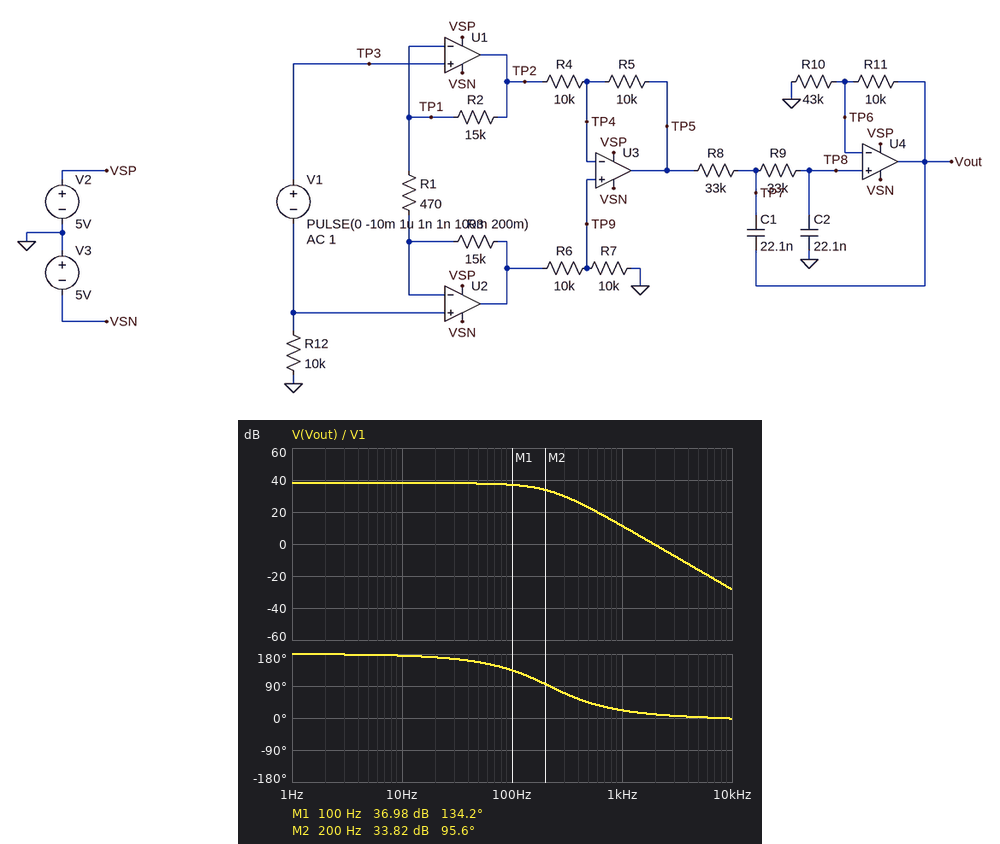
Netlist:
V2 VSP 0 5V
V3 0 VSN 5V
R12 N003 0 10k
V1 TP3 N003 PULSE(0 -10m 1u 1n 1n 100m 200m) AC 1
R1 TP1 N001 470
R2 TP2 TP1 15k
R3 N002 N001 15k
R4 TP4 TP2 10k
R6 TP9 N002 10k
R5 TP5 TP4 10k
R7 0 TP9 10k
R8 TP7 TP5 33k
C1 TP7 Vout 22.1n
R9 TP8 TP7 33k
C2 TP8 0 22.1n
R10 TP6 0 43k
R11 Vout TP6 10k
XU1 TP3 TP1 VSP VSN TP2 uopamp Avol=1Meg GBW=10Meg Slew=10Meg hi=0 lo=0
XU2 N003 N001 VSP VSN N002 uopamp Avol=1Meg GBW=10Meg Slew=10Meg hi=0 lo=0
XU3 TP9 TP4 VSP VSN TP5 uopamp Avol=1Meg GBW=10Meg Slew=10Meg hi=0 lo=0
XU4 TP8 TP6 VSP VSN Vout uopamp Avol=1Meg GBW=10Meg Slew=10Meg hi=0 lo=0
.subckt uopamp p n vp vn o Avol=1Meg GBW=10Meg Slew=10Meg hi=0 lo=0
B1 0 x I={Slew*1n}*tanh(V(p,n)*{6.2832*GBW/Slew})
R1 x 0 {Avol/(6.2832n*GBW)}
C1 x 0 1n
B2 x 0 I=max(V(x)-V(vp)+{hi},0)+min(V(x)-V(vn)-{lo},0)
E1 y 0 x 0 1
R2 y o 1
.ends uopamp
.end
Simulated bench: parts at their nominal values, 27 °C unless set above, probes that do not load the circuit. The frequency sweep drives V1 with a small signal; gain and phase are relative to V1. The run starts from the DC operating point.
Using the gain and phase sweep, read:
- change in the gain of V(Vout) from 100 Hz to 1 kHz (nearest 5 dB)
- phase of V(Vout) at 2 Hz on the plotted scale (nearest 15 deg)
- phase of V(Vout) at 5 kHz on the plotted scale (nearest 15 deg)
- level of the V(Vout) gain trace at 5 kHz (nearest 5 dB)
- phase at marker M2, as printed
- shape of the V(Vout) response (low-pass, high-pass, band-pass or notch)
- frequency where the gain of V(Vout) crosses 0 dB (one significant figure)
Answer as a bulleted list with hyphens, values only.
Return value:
- -25 dB
- 180 deg
- 0 deg
- -15 dB
- 95.6 deg
- low-pass
- 2 kHz
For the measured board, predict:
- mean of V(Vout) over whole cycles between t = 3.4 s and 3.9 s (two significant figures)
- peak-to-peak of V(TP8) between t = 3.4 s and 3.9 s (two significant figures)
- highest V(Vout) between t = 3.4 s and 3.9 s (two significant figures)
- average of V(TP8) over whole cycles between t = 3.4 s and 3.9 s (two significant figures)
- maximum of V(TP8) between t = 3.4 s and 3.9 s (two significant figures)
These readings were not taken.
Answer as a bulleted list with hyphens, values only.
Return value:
- 400 mV
- 650 mV
- 800 mV
- 320 mV
- 650 mV
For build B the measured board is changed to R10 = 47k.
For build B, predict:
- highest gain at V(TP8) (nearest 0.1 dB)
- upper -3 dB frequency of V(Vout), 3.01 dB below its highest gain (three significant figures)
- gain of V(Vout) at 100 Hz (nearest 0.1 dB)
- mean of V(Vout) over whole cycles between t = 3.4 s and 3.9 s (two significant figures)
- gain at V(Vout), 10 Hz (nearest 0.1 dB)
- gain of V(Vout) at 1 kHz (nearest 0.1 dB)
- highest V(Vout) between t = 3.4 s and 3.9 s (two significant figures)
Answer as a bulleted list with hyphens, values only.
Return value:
- 36.2 dB
- 164 Hz
- 36.8 dB
- 390 mV
- 37.9 dB
- 11.2 dB
- 790 mV
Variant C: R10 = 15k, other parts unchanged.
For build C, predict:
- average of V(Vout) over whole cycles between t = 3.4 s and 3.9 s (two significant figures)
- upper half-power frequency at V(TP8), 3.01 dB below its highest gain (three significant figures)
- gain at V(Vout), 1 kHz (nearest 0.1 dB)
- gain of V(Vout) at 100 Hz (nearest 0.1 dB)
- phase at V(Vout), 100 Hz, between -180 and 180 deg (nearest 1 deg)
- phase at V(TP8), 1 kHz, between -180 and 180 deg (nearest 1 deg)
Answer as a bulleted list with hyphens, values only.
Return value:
- 540 mV
- 229 Hz
- 14.3 dB
- 40.7 dB
- 142 deg
- 17 deg
